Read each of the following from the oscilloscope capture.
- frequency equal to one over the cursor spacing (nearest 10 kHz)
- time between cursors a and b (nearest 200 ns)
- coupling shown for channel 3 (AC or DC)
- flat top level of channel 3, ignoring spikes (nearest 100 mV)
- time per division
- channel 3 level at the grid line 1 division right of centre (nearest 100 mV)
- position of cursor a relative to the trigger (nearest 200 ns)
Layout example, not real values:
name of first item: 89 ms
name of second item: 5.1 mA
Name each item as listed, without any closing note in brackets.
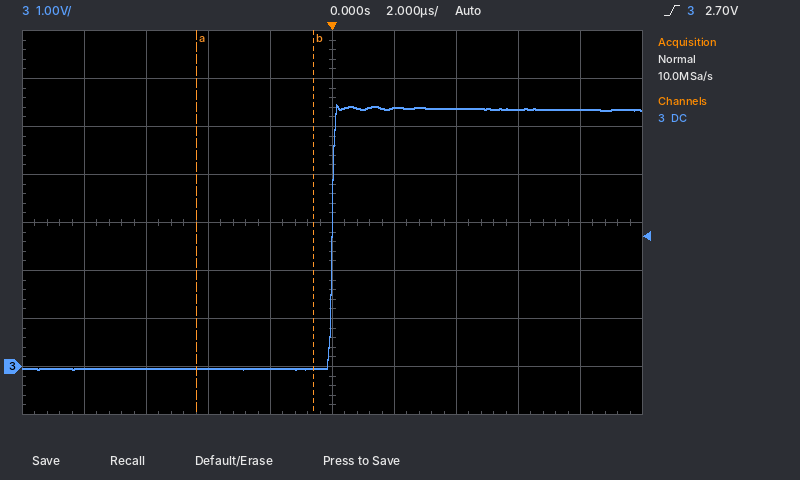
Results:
frequency equal to one over the cursor spacing: 260 kHz
time between cursors a and b: 3.8 µs
coupling shown for channel 3: DC
flat top level of channel 3, ignoring spikes: 5.4 V
time per division: 2 µs
channel 3 level at the grid line 1 division right of centre: 5.4 V
position of cursor a relative to the trigger: -4.4 µs
